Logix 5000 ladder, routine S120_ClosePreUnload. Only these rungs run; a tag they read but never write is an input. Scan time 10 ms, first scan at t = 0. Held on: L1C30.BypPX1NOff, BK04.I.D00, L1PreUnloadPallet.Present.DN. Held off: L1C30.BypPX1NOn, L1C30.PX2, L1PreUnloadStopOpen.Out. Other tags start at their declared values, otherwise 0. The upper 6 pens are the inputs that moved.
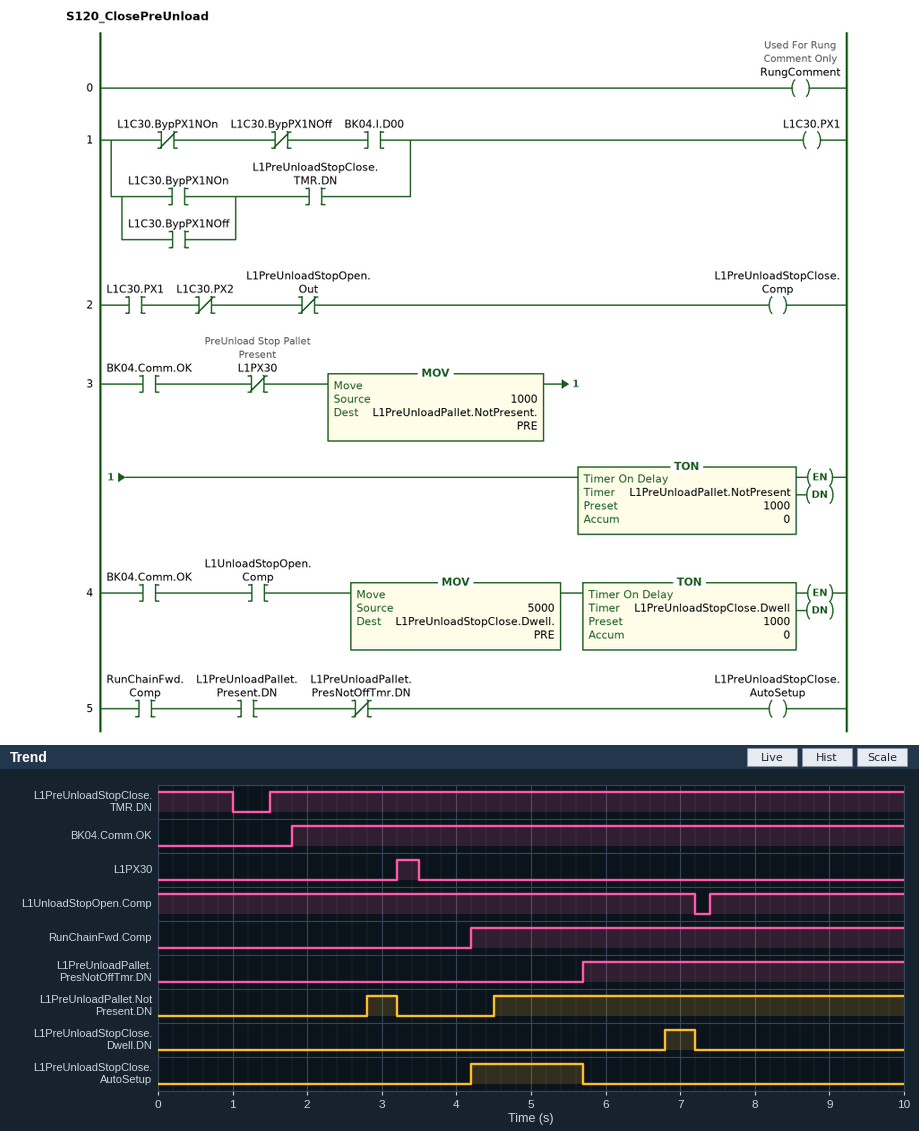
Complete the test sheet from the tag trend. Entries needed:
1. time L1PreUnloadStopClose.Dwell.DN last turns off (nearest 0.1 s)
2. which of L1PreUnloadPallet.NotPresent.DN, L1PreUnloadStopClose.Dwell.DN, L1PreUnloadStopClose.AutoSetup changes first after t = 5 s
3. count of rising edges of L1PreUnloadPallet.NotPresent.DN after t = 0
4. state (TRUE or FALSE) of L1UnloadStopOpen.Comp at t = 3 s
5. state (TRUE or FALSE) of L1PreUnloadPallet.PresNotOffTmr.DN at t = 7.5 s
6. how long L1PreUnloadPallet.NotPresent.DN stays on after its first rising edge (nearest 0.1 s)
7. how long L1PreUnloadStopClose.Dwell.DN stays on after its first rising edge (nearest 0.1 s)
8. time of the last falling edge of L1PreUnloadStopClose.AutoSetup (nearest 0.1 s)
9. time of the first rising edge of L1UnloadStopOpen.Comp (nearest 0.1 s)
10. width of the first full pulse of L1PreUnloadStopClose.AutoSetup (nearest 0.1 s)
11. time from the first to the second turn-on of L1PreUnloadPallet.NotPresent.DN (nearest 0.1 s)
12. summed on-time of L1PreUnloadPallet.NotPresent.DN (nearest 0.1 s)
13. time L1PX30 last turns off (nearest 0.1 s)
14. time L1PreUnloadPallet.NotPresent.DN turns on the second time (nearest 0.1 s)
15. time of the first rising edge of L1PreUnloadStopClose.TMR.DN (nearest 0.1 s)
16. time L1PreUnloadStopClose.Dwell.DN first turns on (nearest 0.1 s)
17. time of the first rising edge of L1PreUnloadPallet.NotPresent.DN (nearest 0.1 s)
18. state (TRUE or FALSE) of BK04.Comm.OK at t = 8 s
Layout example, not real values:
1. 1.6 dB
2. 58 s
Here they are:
1. 7.2 s
2. L1PreUnloadStopClose.AutoSetup
3. 2
4. TRUE
5. TRUE
6. 0.4 s
7. 0.4 s
8. 5.7 s
9. 7.4 s
10. 1.5 s
11. 1.7 s
12. 5.9 s
13. 3.5 s
14. 4.5 s
15. 1.5 s
16. 6.8 s
17. 2.8 s
18. TRUE
